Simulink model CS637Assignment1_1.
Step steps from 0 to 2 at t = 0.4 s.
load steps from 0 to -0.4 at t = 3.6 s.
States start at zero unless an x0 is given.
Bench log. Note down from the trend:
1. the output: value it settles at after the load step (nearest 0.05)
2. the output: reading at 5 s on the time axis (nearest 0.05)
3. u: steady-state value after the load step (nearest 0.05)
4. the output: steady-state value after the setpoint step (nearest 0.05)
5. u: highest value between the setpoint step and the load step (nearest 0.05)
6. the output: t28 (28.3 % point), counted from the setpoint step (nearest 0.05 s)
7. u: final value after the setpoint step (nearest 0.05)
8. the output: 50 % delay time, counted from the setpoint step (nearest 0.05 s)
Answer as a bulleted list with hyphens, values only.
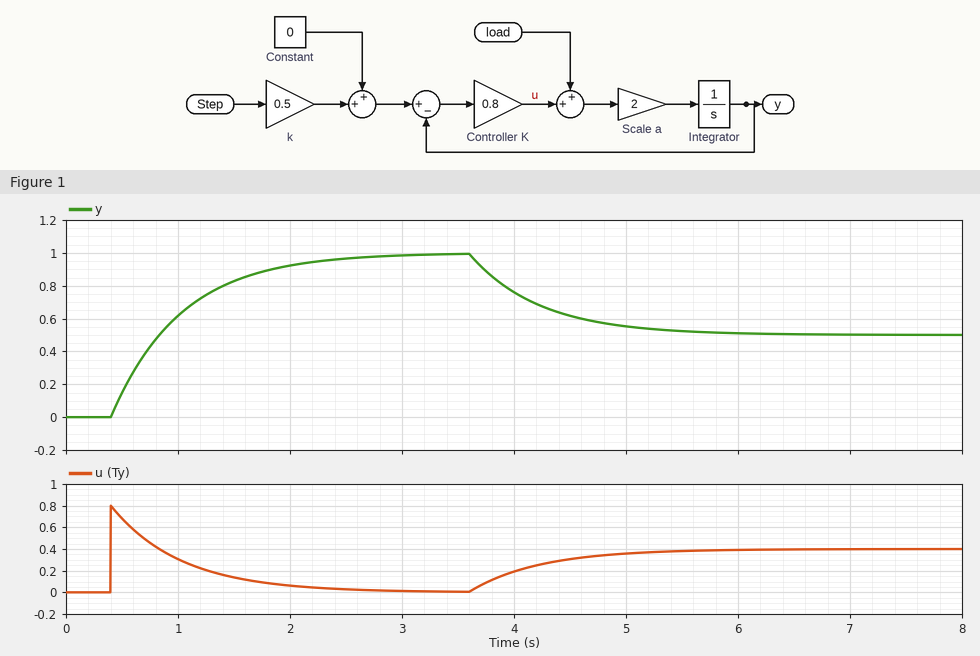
- 0.50
- 0.55
- 0.40
- 1.00
- 0.80
- 0.20 s
- 0.00
- 0.45 s
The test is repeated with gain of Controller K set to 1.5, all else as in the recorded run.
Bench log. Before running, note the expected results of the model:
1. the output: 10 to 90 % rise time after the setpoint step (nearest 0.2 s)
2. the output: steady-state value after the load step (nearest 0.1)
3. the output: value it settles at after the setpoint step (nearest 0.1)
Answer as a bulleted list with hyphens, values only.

- 0.8 s
- 0.7
- 1.0
